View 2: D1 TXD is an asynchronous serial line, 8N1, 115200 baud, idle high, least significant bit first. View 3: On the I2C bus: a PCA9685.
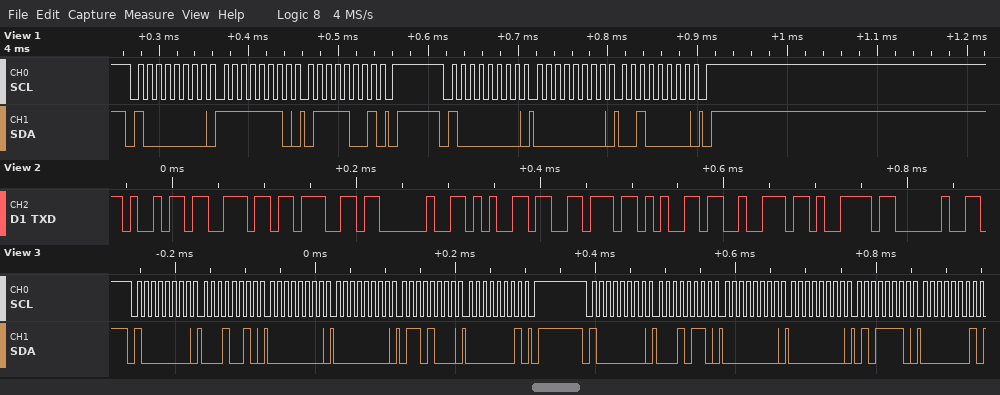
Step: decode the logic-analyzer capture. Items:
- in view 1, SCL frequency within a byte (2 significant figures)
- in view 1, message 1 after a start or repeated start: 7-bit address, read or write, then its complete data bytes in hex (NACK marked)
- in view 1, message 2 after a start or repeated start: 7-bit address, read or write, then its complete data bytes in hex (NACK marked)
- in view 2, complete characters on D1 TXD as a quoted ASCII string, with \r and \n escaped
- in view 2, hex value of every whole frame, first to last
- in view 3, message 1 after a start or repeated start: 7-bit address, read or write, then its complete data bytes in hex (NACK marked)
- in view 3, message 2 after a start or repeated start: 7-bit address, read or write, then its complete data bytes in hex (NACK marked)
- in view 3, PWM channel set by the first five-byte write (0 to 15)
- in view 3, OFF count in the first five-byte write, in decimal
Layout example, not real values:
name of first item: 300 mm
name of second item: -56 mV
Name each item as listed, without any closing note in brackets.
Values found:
in view 1, SCL frequency within a byte: 100 kHz
in view 1, message 1 after a start or repeated start: 7-bit address, read or write, then its complete data bytes in hex: 0x40 write: FE 79
in view 1, message 2 after a start or repeated start: 7-bit address, read or write, then its complete data bytes in hex: 0x40 write: 00 20
in view 2, complete characters on D1 TXD as a quoted ASCII string, with \r and \n escaped: "ing every "
in view 2, hex value of every whole frame, first to last: 69 6E 67 20 65 76 65 72 79 20
in view 3, message 1 after a start or repeated start: 7-bit address, read or write, then its complete data bytes in hex: 0x40 write: 12 00 00 68 01
in view 3, message 2 after a start or repeated start: 7-bit address, read or write, then its complete data bytes in hex: 0x40 write: 16 00 00 5E 01
in view 3, PWM channel set by the first five-byte write: 3
in view 3, OFF count in the first five-byte write, in decimal: 360
